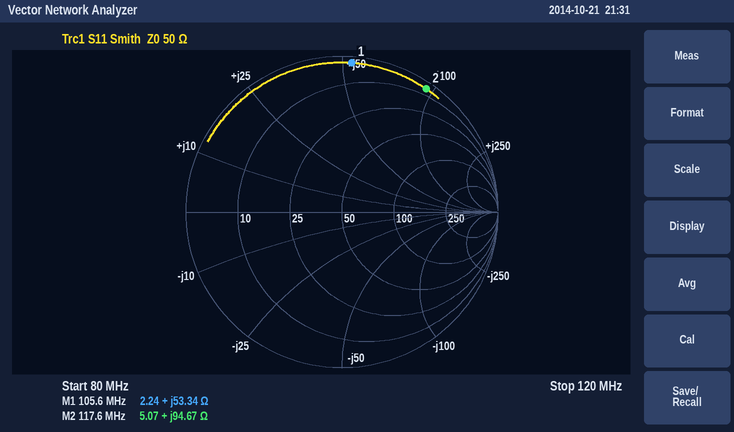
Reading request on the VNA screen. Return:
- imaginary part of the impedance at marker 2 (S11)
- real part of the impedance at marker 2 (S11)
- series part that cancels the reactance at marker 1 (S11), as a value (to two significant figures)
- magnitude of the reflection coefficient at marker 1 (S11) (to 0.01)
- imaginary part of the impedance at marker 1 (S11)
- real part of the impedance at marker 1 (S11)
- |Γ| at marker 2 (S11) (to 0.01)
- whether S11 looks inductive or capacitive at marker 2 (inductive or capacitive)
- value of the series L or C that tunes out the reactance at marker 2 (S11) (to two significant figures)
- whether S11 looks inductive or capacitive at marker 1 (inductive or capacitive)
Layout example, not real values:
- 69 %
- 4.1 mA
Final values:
- +94.67 Ω
- 5.07 Ω
- 28 pF
- 0.96
- +53.34 Ω
- 2.24 Ω
- 0.96
- inductive
- 14 pF
- inductive
